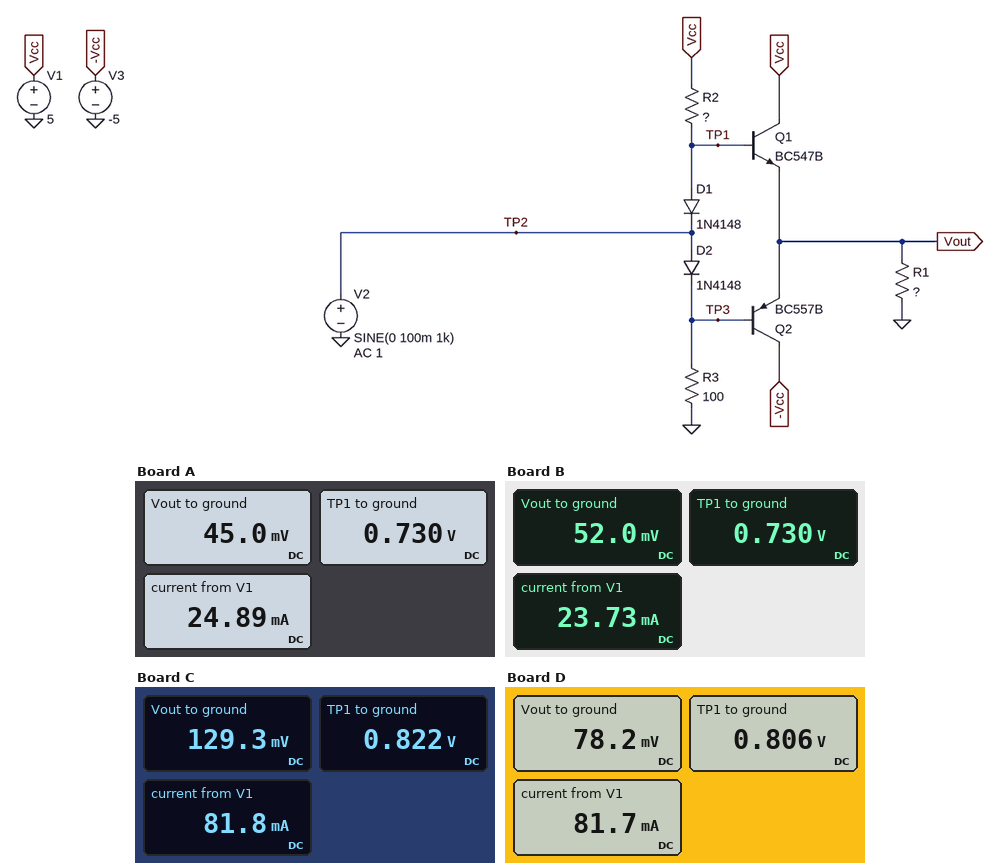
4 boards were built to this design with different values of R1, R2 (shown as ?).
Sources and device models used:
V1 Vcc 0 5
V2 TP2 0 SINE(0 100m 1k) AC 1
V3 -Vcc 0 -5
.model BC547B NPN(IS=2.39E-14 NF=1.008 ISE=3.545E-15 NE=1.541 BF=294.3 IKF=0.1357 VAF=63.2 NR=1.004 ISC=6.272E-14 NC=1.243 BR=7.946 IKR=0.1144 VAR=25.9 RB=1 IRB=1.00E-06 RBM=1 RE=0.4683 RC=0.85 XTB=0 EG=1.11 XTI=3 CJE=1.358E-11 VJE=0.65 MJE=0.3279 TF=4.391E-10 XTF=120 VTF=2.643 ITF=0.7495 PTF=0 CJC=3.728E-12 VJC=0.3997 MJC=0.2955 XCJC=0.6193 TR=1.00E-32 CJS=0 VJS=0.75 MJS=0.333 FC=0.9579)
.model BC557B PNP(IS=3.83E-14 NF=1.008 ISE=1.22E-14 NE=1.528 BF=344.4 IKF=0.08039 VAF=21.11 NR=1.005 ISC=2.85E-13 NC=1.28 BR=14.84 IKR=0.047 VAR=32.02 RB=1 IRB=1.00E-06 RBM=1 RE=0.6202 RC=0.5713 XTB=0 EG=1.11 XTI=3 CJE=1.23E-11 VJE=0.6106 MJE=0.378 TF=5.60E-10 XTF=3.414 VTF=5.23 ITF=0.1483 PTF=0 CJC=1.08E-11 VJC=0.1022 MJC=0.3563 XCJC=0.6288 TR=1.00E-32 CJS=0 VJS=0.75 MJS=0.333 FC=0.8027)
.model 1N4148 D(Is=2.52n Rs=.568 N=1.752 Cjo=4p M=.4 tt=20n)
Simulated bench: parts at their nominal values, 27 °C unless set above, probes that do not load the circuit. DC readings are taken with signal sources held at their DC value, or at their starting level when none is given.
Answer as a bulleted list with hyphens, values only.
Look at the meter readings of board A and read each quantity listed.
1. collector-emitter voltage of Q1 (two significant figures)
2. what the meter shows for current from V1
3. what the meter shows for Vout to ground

- 5.0 V
- 24.89 mA
- 45.0 mV
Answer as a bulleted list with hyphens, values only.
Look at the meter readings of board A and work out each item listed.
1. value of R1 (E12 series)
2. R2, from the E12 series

- 8.2 Ω
- 220 Ω
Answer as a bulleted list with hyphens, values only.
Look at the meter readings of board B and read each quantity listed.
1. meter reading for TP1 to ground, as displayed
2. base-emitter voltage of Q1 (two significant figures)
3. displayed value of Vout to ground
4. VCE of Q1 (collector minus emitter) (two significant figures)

- 0.730 V
- 680 mV
- 52.0 mV
- 4.9 V
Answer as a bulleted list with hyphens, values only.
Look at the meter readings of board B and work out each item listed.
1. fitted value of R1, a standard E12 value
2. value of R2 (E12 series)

- 12 Ω
- 220 Ω
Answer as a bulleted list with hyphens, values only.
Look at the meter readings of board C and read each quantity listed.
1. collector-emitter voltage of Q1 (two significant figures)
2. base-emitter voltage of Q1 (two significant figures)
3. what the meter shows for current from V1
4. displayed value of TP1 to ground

- 4.9 V
- 690 mV
- 81.8 mA
- 0.822 V
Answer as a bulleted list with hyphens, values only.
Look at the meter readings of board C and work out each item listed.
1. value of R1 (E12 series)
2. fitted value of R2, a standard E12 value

- 18 Ω
- 56 Ω
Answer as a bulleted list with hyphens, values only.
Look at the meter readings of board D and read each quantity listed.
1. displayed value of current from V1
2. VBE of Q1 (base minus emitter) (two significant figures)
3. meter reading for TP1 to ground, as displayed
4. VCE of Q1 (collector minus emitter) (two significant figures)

- 81.7 mA
- 730 mV
- 0.806 V
- 4.9 V
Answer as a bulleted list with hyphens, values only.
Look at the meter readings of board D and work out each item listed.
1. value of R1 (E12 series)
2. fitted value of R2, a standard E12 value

- 3.9 Ω
- 68 Ω
